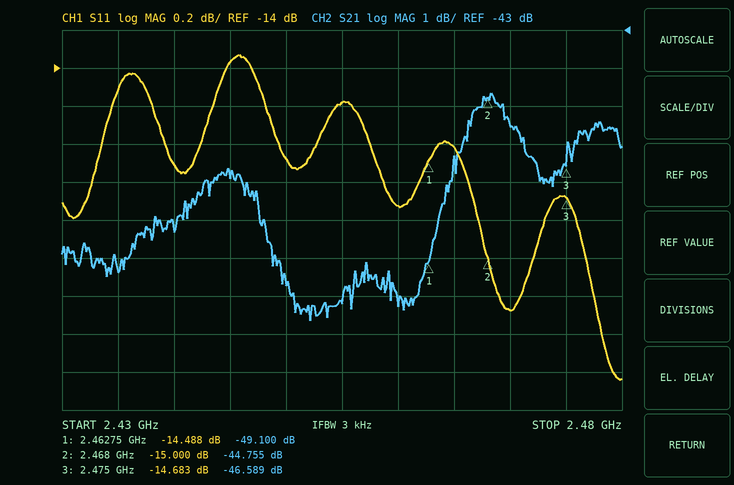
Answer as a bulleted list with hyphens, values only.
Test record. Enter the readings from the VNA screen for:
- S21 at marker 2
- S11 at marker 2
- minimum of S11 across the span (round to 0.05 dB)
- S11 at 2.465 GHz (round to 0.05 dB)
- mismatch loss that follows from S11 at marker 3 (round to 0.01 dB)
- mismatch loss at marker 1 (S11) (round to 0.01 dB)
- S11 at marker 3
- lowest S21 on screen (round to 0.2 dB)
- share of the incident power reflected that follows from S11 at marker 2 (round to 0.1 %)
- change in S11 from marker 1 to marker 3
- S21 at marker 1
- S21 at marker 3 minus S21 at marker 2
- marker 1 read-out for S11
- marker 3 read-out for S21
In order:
- -44.755 dB
- -15.000 dB
- -15.65 dB
- -14.40 dB
- 0.15 dB
- 0.16 dB
- -14.683 dB
- -50.6 dB
- 3.2 %
- -0.195 dB
- -49.100 dB
- -1.834 dB
- -14.488 dB
- -46.589 dB
